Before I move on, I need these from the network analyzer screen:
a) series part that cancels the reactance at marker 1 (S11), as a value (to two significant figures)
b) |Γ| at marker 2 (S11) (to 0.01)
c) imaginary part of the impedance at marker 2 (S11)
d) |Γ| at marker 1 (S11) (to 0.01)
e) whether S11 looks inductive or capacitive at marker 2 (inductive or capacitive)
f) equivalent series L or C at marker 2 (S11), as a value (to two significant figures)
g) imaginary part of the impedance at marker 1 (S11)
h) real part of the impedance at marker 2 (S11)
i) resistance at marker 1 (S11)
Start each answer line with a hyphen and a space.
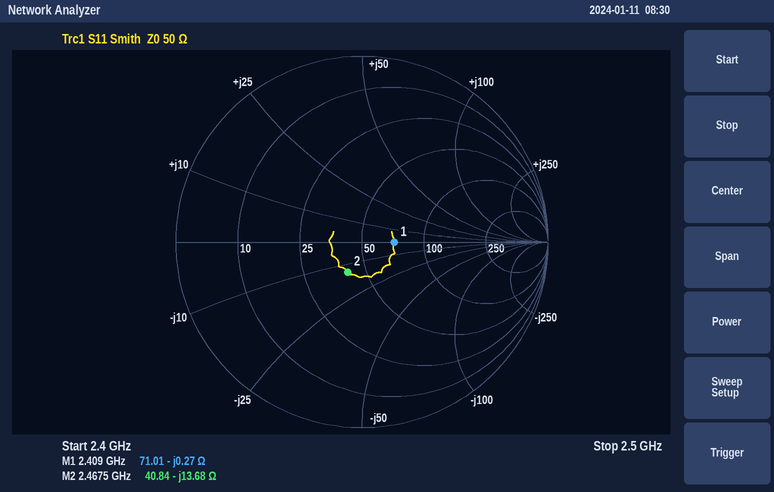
- 18 pH
- 0.18
- -13.68 Ω
- 0.17
- capacitive
- 4.7 pF
- -0.27 Ω
- 40.84 Ω
- 71.01 Ω
